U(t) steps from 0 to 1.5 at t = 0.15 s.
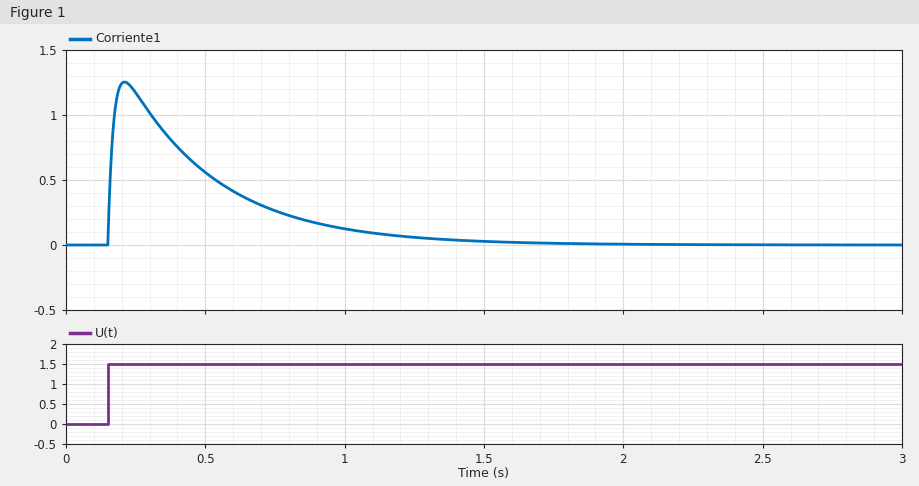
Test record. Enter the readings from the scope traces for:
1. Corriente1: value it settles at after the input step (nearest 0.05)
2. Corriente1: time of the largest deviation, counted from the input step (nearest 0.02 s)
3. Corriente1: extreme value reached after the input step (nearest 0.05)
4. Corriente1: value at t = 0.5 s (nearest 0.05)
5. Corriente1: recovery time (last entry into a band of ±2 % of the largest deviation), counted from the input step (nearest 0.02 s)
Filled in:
0.00
0.06 s
1.25
0.55
1.38 s
